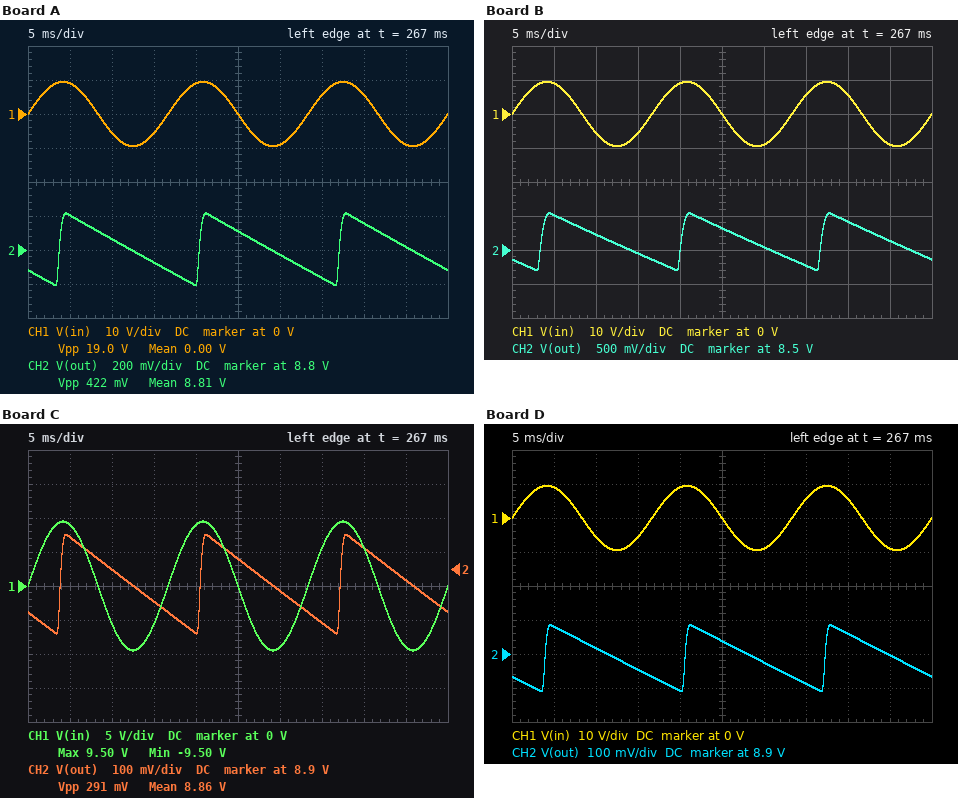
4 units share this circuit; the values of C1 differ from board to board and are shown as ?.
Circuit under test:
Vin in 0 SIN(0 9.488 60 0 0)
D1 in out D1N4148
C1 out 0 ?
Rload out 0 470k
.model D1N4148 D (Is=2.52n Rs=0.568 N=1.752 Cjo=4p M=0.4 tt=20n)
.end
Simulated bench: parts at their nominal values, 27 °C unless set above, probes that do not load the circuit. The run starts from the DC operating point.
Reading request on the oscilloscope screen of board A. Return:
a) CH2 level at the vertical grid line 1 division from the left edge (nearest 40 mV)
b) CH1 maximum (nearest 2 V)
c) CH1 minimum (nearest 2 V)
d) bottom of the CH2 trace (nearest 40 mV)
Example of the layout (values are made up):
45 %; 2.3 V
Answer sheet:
9.00 V; 10 V; -10 V; 8.60 V
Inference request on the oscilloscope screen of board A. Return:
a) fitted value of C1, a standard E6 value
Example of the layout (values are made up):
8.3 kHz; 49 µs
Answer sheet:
680 nF
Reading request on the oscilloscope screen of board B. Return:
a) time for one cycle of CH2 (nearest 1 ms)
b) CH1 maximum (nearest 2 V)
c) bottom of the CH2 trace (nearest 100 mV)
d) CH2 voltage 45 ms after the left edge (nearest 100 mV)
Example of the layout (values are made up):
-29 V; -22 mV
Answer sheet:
17 ms; 10 V; 8.2 V; 8.6 V
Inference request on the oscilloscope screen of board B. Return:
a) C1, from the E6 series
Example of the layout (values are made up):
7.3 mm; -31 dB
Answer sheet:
330 nF
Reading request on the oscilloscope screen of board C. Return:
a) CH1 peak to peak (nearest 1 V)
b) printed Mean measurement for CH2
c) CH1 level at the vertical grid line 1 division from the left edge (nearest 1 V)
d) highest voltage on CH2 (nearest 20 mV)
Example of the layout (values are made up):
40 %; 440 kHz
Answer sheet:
19 V; 8.86 V; 9 V; 9.00 V
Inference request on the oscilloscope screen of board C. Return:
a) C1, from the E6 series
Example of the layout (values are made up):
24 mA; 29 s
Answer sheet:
1 µF
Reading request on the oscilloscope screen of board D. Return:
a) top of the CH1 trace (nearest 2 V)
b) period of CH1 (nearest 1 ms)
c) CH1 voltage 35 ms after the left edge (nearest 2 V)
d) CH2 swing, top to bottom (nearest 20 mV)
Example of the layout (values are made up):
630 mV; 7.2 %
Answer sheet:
10 V; 17 ms; 6 V; 200 mV
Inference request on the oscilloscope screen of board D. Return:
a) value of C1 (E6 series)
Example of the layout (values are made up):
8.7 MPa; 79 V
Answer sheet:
1.5 µF
